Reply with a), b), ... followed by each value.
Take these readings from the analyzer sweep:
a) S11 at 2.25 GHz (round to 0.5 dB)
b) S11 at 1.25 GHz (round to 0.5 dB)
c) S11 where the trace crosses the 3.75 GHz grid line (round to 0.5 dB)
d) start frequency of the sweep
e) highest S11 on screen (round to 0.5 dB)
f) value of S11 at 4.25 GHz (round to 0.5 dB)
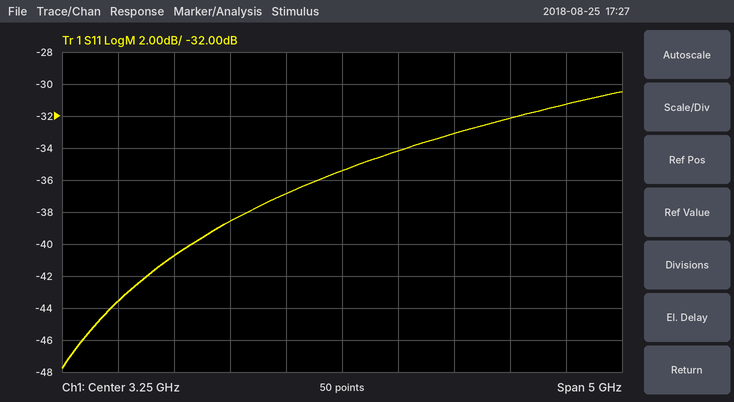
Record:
a) -38.5 dB
b) -43.5 dB
c) -34.0 dB
d) 750 MHz
e) -30.5 dB
f) -33.0 dB
